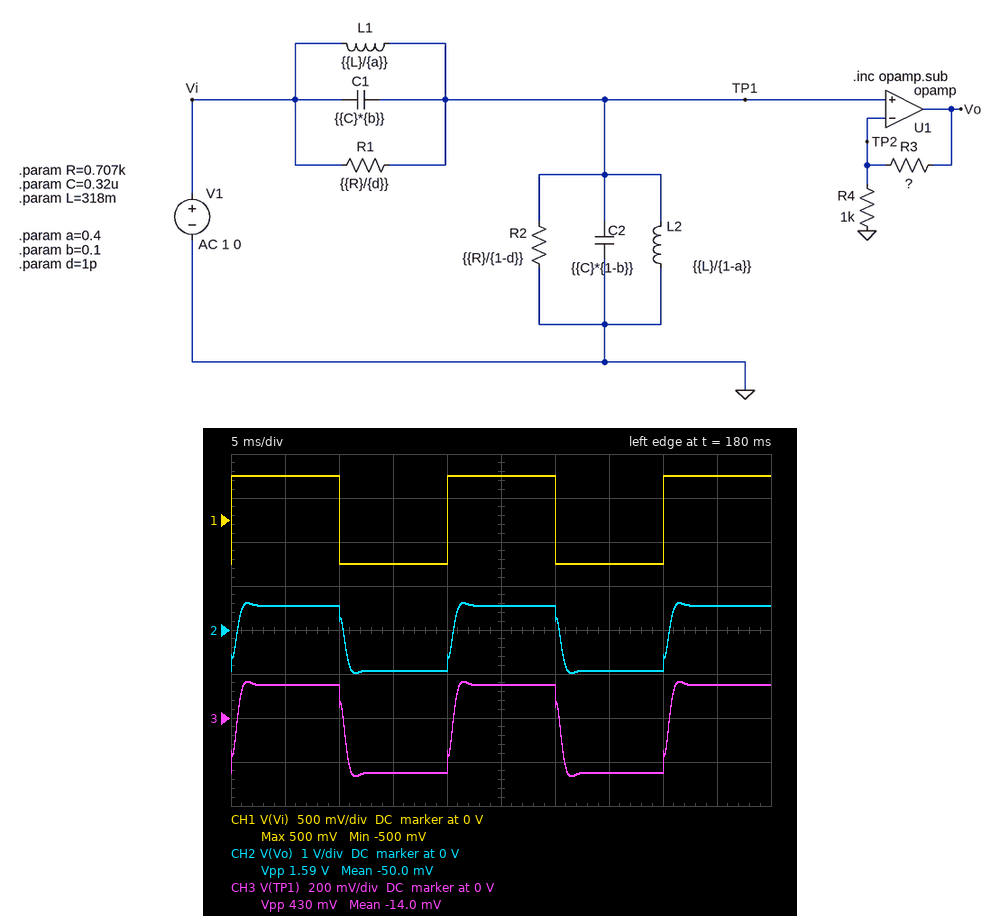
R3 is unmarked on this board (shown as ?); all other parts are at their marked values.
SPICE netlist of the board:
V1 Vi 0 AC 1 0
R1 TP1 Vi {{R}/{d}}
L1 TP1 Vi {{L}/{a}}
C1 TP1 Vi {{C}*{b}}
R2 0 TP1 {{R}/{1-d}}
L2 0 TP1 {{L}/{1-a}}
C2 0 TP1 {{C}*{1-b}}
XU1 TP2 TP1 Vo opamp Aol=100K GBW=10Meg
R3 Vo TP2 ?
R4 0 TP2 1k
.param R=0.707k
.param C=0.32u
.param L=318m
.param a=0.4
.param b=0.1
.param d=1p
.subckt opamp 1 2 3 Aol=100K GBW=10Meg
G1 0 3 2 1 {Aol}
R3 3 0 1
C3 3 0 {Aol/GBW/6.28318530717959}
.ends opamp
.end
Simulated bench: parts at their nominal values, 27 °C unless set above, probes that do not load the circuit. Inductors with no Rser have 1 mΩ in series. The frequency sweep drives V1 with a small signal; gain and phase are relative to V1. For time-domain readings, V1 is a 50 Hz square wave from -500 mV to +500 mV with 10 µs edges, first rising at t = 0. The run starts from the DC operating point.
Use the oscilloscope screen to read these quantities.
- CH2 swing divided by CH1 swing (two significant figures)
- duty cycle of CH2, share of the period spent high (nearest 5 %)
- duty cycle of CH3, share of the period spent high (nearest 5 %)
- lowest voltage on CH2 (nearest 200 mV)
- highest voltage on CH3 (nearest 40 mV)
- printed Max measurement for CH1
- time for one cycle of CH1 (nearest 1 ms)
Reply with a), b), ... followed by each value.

a) 1.6
b) 50 %
c) 50 %
d) -1.0 V
e) 160 mV
f) 500 mV
g) 20 ms
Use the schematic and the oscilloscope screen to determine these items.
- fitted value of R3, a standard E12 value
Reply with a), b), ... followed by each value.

a) 2.7 kΩ
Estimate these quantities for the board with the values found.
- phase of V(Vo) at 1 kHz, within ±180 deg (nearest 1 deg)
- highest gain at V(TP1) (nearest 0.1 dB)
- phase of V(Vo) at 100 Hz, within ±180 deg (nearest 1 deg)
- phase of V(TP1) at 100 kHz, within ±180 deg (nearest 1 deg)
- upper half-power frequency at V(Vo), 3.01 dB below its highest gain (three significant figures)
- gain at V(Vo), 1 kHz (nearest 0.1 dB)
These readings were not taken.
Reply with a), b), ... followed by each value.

a) 43 deg
b) -8.0 dB
c) -16 deg
d) 0 deg
e) 400 Hz
f) -56.2 dB
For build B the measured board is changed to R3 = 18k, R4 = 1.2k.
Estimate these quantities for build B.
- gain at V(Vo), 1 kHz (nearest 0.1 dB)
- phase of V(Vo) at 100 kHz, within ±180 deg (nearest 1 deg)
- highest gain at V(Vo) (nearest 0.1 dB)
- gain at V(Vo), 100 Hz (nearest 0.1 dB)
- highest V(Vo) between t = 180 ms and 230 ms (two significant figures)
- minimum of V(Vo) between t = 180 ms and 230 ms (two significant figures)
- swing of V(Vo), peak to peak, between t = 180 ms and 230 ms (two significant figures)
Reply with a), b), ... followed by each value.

a) -43.5 dB
b) -9 deg
c) 16.1 dB
d) 16.0 dB
e) 2.6 V
f) -4.2 V
g) 6.9 V
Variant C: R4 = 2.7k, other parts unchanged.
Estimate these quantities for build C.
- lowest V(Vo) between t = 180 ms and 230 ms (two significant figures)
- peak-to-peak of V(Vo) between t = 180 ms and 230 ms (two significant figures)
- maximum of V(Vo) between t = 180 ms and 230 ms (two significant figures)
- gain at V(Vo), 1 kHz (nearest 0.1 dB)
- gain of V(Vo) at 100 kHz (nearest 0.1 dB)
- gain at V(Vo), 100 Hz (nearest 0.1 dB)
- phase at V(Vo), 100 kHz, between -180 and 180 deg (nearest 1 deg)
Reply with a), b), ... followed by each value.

a) -530 mV
b) 860 mV
c) 330 mV
d) -61.5 dB
e) -14.0 dB
f) -2.0 dB
g) -1 deg
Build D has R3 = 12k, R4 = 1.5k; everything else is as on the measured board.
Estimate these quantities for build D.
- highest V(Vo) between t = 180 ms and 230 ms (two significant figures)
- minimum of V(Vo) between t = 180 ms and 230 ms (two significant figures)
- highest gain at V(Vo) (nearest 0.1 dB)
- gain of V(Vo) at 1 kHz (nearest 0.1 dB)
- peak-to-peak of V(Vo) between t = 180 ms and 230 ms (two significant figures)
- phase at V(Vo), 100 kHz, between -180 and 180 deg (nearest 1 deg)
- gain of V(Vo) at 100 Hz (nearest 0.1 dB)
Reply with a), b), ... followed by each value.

a) 1.5 V
b) -2.4 V
c) 11.1 dB
d) -48.5 dB
e) 3.9 V
f) -5 deg
g) 11.0 dB
